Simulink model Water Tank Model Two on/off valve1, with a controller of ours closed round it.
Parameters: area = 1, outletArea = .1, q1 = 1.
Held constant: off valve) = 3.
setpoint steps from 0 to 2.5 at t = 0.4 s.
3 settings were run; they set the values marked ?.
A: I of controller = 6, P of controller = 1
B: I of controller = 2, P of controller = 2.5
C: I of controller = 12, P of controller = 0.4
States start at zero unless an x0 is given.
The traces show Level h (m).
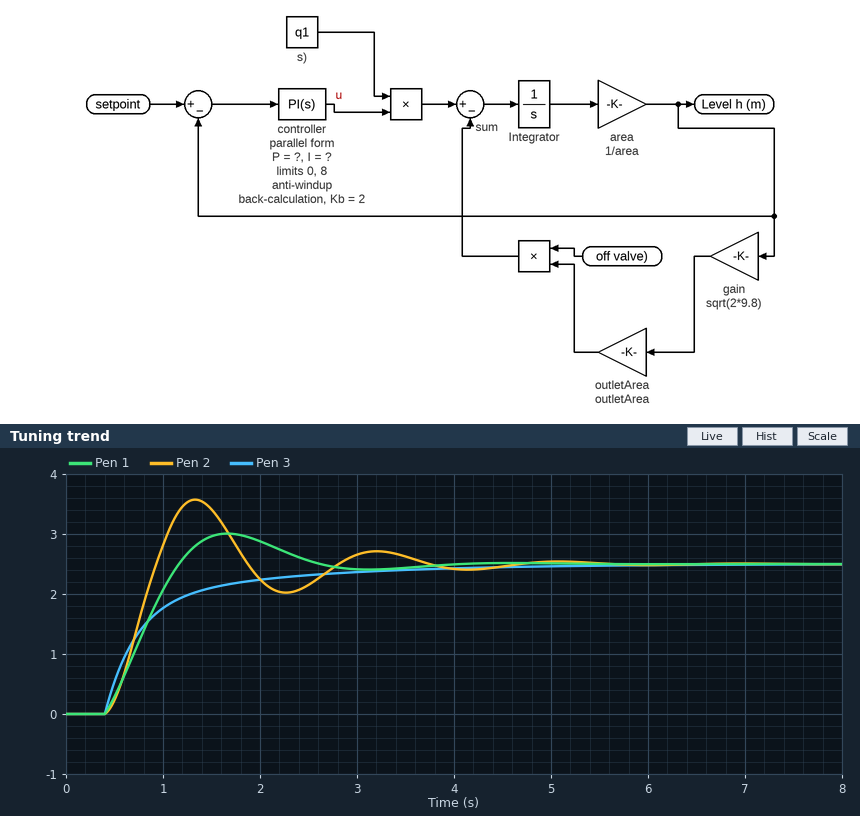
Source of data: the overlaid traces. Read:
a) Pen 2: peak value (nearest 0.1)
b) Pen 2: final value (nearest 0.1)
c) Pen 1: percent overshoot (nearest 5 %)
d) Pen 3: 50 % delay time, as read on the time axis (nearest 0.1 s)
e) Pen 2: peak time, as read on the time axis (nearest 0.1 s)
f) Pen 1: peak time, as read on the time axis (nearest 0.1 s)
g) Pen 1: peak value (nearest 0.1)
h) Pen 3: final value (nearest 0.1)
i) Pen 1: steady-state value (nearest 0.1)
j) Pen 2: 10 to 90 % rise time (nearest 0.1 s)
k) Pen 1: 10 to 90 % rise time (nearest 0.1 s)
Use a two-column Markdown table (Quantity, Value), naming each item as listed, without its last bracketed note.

| Quantity | Value |
|---|---|
| Pen 2: peak value | 3.6 |
| Pen 2: final value | 2.5 |
| Pen 1: percent overshoot | 20 % |
| Pen 3: 50 % delay time, as read on the time axis | 0.7 s |
| Pen 2: peak time, as read on the time axis | 1.3 s |
| Pen 1: peak time, as read on the time axis | 1.7 s |
| Pen 1: peak value | 3.0 |
| Pen 3: final value | 2.5 |
| Pen 1: steady-state value | 2.5 |
| Pen 2: 10 to 90 % rise time | 0.4 s |
| Pen 1: 10 to 90 % rise time | 0.6 s |
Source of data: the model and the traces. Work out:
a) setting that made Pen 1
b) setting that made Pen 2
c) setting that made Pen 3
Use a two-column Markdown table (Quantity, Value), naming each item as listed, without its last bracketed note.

| Quantity | Value |
|---|---|
| setting that made Pen 1 | A |
| setting that made Pen 2 | C |
| setting that made Pen 3 | B |
